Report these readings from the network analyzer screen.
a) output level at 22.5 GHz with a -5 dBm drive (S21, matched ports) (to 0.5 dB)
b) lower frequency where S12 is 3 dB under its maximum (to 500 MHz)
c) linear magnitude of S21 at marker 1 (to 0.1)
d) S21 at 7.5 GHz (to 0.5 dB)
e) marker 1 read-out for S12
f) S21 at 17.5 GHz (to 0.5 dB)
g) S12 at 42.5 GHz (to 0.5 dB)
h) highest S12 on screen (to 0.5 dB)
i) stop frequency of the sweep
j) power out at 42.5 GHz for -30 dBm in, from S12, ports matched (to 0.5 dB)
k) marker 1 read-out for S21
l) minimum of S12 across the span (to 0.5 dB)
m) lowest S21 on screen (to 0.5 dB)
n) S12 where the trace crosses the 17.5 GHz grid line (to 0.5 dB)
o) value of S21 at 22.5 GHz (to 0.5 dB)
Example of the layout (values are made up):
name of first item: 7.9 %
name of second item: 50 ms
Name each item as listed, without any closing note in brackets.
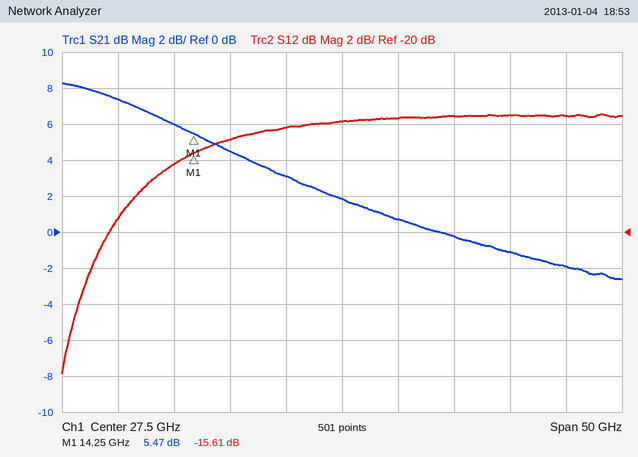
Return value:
output level at 22.5 GHz with a -5 dBm drive (S21, matched ports): -2.0 dBm
lower frequency where S12 is 3 dB under its maximum: 12.0 GHz
linear magnitude of S21 at marker 1: 1.9
S21 at 7.5 GHz: 7.5 dB
marker 1 read-out for S12: -15.61 dB
S21 at 17.5 GHz: 4.5 dB
S12 at 42.5 GHz: -13.5 dB
highest S12 on screen: -13.5 dB
stop frequency of the sweep: 52.5 GHz
power out at 42.5 GHz for -30 dBm in, from S12, ports matched: -43.5 dBm
marker 1 read-out for S21: 5.47 dB
minimum of S12 across the span: -28.0 dB
lowest S21 on screen: -2.5 dB
S12 where the trace crosses the 17.5 GHz grid line: -15.0 dB
value of S21 at 22.5 GHz: 3.0 dB
